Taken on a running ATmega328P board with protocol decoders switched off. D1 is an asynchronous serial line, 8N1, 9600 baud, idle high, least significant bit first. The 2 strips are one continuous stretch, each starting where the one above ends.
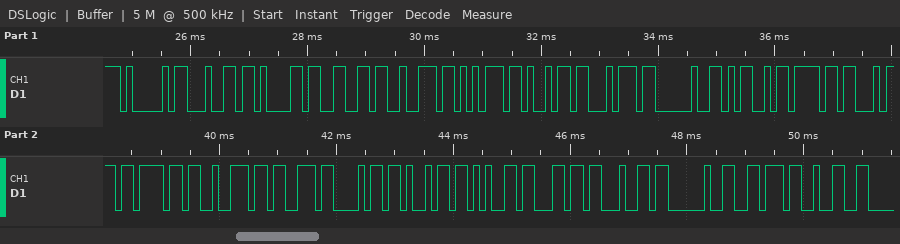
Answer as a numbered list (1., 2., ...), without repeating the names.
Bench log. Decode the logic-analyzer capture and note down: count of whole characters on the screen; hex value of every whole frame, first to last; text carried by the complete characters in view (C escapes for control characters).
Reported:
1. 23
2. 0x41 0x64 0x61 0x66 0x72 0x75 0x69 0x74 0x20 0x4D 0x6F 0x74 0x6F 0x72 0x73 0x68 0x69 0x65 0x6C 0x64 0x20 0x76 0x32
3. "Adafruit Motorshield v2"
